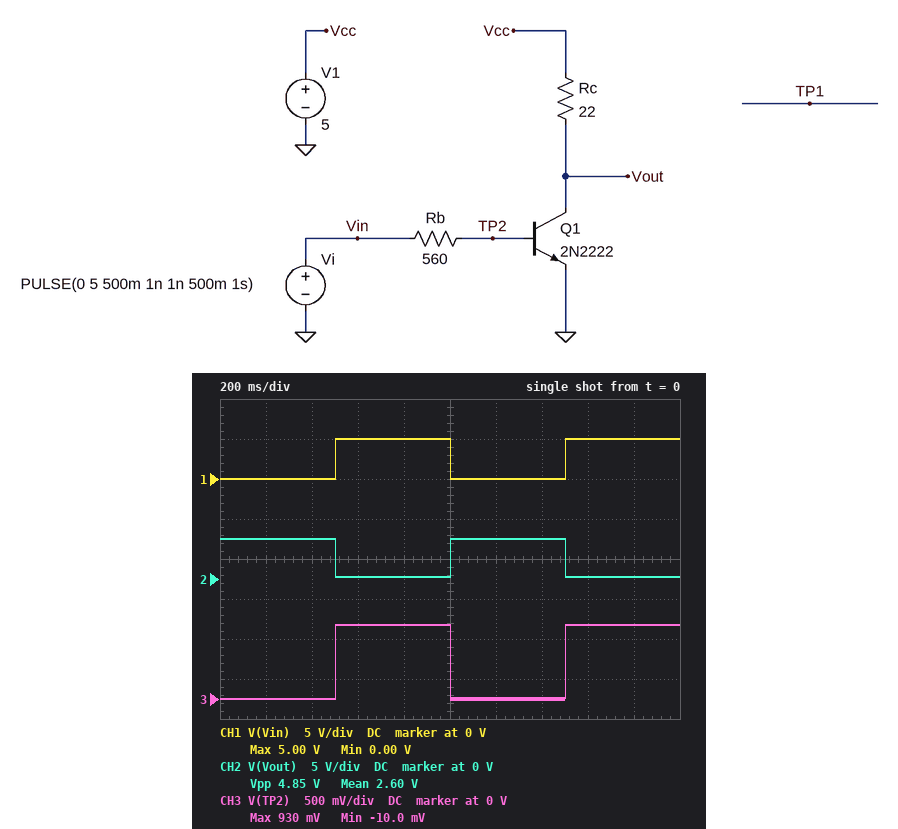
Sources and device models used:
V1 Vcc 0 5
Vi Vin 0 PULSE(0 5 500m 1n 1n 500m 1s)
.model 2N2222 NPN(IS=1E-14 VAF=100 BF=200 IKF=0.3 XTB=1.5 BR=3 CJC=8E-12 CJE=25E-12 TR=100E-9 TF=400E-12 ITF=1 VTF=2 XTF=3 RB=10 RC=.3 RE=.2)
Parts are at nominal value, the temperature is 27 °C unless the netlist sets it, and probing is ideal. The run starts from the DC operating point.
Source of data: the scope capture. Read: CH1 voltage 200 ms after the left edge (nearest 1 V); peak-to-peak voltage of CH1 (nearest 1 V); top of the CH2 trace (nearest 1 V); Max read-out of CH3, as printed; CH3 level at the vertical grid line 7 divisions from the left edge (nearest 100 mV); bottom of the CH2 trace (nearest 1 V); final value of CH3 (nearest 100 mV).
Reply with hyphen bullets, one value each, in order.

- 0 V
- 5 V
- 5 V
- 930 mV
- 0 V
- 0 V
- 900 mV
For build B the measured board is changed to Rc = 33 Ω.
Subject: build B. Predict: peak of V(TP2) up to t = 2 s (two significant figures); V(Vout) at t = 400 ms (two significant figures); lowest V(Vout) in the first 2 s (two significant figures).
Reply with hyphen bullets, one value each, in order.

- 900 mV
- 5.0 V
- 140 mV
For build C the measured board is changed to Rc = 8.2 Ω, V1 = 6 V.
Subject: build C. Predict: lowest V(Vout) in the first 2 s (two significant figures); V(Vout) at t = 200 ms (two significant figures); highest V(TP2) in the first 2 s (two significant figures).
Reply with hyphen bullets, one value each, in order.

- 1.7 V
- 6.0 V
- 1.0 V
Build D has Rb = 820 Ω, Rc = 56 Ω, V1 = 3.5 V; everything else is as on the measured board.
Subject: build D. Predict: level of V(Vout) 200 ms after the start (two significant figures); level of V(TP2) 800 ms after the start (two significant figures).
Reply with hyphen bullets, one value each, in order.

- 3.5 V
- 840 mV
